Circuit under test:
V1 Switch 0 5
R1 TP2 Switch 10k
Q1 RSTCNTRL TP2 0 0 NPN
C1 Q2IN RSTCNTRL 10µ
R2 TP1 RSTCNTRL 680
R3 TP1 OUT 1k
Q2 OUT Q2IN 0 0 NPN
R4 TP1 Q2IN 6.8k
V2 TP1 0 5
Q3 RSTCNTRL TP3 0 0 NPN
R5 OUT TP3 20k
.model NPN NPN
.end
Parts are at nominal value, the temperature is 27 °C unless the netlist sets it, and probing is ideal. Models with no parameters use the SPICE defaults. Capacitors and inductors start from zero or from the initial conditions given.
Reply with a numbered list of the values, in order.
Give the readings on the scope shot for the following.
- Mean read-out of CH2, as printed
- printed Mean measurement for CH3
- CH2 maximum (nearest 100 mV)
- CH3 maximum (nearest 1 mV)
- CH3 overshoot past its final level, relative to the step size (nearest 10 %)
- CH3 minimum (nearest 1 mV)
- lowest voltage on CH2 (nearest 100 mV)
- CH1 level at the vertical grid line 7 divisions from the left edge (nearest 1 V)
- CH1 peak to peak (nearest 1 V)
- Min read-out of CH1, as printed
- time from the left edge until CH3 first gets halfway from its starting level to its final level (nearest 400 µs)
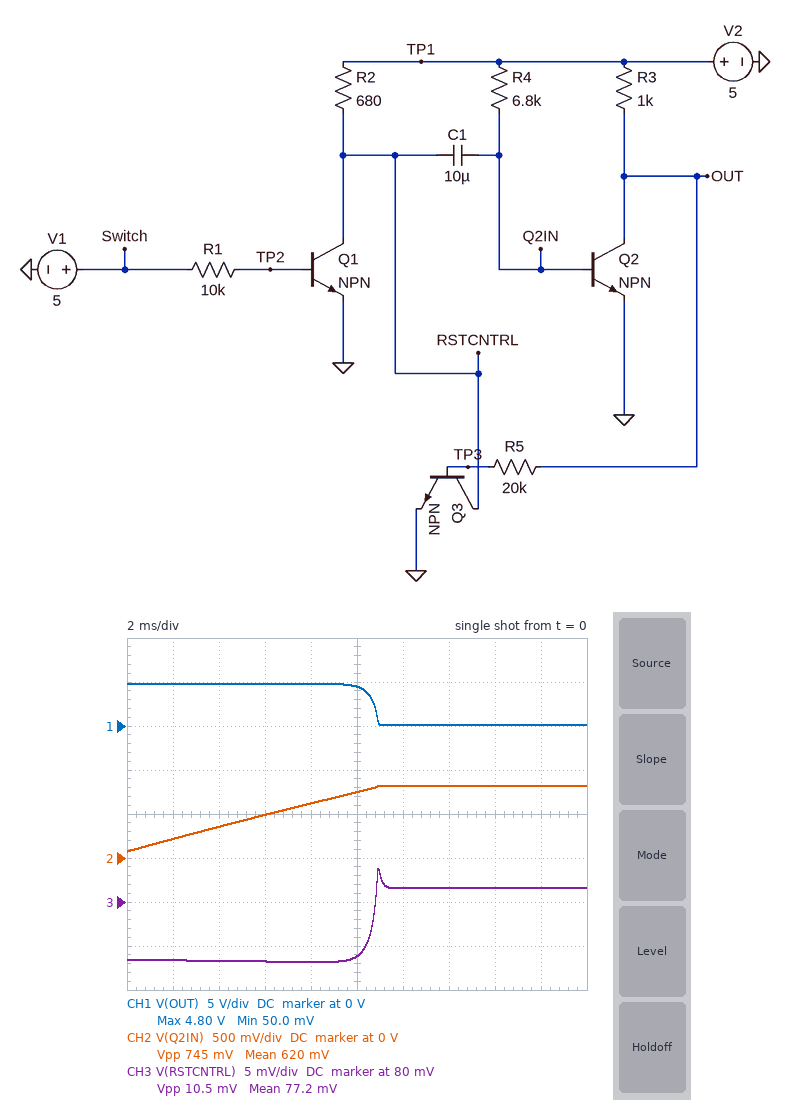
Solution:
1. 620 mV
2. 77.2 mV
3. 800 mV
4. 84 mV
5. 30 %
6. 73 mV
7. 100 mV
8. 0 V
9. 5 V
10. 50.0 mV
11. 10.8 ms
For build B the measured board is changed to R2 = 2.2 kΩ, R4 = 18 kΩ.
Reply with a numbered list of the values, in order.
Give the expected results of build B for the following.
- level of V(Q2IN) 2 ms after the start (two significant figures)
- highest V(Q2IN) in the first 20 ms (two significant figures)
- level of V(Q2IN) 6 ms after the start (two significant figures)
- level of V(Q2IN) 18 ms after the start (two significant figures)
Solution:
1. 100 mV
2. 570 mV
3. 210 mV
4. 520 mV
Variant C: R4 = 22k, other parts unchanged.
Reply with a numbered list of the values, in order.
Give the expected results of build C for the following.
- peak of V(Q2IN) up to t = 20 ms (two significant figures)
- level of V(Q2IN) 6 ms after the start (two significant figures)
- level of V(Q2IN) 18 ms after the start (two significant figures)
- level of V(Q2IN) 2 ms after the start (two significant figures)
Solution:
1. 500 mV
2. 200 mV
3. 460 mV
4. 120 mV
